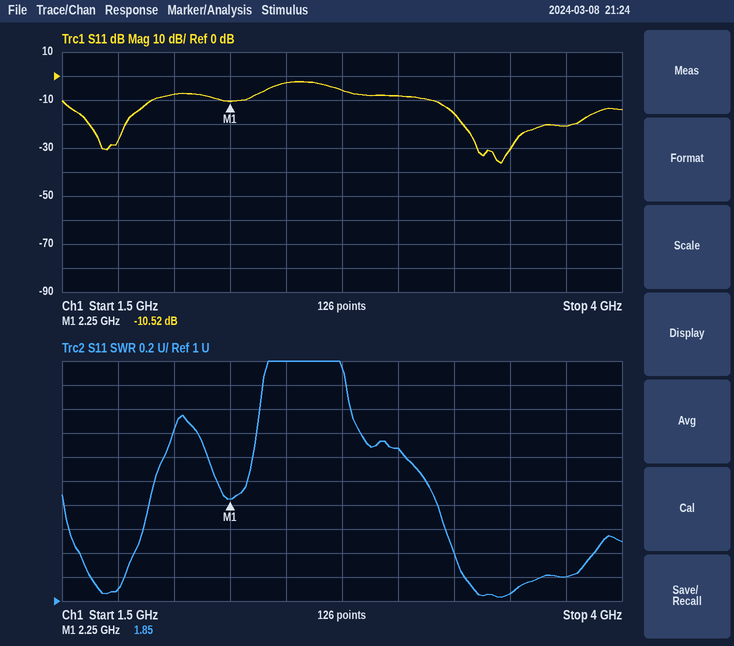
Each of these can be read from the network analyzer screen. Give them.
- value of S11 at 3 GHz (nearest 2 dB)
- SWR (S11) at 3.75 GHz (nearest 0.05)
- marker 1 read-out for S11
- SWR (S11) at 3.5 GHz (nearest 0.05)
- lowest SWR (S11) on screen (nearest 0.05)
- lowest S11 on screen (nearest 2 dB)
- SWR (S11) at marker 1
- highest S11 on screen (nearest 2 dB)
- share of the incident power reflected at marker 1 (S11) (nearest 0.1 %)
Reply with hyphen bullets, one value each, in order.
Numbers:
- -8 dB
- 1.20
- -10.52 dB
- 1.05
- 1.05
- -36 dB
- 1.85
- -2 dB
- 8.9 %
